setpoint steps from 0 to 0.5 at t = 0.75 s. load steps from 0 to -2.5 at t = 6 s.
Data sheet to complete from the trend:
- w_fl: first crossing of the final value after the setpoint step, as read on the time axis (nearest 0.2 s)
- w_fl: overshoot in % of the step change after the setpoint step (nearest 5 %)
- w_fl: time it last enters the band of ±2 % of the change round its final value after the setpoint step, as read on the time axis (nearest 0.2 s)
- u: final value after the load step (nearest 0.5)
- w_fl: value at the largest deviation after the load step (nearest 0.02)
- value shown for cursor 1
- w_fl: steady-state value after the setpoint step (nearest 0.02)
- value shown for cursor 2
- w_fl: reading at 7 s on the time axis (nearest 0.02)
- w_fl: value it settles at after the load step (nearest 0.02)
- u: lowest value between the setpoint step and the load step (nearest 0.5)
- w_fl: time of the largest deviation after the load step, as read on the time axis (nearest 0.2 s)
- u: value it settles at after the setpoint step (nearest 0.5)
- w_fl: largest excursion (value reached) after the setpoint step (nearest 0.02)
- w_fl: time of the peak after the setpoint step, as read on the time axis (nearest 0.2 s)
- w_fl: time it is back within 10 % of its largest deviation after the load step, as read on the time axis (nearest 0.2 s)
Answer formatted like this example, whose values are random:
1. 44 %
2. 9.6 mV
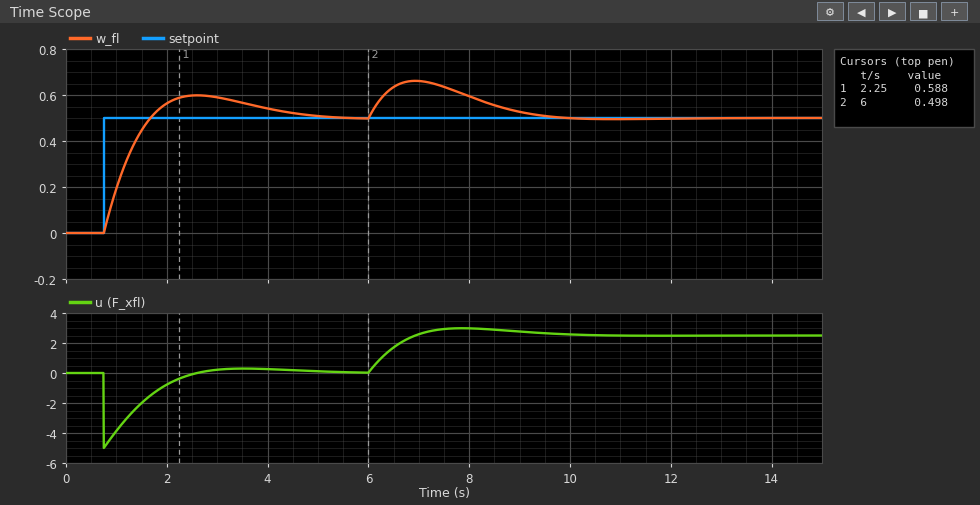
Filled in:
1. 1.6 s
2. 20 %
3. 5.0 s
4. 2.5
5. 0.66
6. 0.588
7. 0.50
8. 0.498
9. 0.66
10. 0.50
11. -5.0
12. 7.0 s
13. 0.0
14. 0.60
15. 2.6 s
16. 9.2 s
